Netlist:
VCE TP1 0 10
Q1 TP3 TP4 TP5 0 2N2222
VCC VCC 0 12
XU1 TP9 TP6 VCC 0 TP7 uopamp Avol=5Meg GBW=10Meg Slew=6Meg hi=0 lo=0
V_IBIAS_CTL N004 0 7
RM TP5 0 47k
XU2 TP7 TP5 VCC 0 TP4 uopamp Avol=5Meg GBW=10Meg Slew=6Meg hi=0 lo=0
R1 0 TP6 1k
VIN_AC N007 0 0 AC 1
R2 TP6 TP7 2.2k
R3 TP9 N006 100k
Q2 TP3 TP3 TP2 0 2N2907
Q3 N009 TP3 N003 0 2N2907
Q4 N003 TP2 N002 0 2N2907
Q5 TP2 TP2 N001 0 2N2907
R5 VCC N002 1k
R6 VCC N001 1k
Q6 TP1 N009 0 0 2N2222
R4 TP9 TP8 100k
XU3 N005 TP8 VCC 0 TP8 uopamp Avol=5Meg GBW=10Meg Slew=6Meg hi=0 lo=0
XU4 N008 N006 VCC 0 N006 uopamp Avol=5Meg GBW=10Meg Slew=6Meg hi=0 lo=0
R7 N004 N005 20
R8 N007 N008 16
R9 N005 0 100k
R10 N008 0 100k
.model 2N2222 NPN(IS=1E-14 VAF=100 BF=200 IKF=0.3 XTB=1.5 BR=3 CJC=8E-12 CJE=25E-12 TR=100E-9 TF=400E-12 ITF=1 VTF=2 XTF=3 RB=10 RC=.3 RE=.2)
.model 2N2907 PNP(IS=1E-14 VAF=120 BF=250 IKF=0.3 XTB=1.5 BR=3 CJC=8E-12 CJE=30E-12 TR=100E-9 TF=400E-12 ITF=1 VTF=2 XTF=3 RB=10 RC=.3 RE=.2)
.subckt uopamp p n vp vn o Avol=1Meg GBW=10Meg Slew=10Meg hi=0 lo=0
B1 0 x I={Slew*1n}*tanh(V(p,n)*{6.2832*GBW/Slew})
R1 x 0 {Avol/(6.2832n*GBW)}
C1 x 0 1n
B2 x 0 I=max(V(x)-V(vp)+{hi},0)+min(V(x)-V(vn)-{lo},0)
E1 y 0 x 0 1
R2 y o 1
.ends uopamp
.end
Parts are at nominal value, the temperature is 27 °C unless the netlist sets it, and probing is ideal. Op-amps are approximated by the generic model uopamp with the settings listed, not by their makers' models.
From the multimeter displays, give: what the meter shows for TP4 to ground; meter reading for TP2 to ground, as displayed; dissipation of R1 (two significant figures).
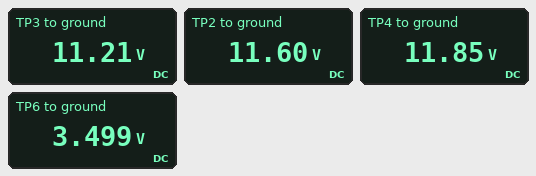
11.85 V
11.60 V
12 mW
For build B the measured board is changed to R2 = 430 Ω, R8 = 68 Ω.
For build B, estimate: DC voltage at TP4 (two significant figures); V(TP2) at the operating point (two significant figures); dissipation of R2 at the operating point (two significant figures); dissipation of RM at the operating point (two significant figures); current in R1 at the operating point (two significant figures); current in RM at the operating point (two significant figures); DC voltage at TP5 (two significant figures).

5.6 V
11 V
5.3 mW
530 µW
3.5 mA
110 µA
5.0 V
